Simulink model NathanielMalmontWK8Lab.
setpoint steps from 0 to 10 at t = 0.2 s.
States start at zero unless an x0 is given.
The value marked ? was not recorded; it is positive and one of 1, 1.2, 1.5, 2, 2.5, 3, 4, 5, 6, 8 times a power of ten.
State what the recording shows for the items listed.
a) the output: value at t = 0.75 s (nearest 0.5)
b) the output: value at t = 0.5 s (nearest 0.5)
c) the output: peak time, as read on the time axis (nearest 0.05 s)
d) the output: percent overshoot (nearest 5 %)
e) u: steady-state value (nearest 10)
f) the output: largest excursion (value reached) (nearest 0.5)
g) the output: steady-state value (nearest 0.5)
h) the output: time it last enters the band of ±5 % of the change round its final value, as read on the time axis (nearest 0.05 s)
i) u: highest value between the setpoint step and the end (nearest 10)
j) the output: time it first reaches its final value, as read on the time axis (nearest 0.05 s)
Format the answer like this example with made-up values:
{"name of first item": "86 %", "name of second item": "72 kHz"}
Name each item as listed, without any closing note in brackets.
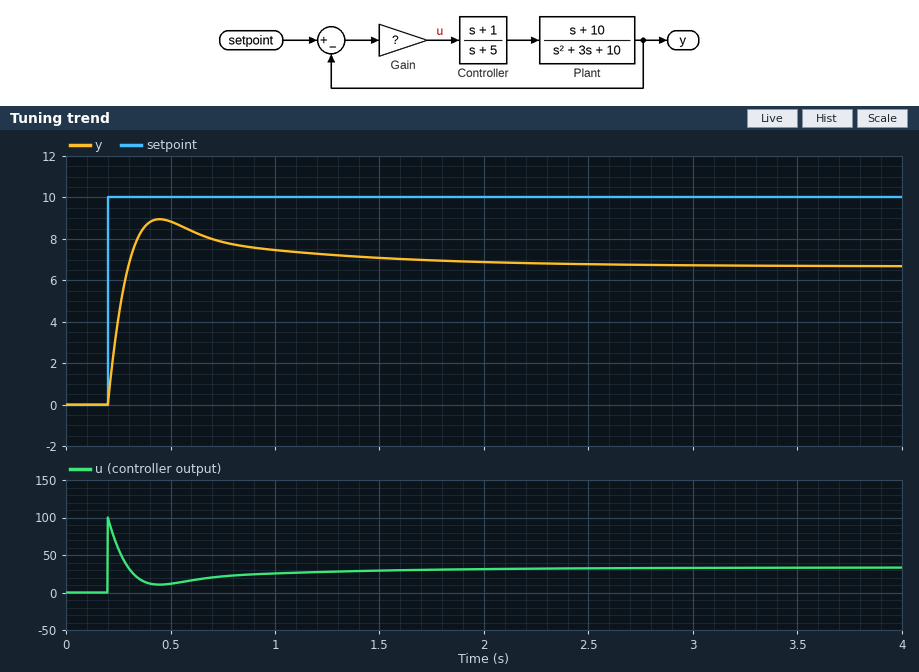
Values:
{"the output: value at t = 0.75 s": "8.0", "the output: value at t = 0.5 s": "9.0", "the output: peak time, as read on the time axis": "0.45 s", "the output: percent overshoot": "35 %", "u: steady-state value": "30", "the output: largest excursion (value reached)": "9.0", "the output: steady-state value": "6.5", "the output: time it last enters the band of ±5 % of the change round its final value, as read on the time axis": "1.65 s", "u: highest value between the setpoint step and the end": "100", "the output: time it first reaches its final value, as read on the time axis": "0.30 s"}
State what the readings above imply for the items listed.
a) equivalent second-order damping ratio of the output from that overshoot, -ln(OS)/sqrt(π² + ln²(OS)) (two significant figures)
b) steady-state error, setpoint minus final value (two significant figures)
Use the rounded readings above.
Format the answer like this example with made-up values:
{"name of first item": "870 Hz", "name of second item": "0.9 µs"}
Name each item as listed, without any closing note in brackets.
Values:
{"equivalent second-order damping ratio of the output from that overshoot, -ln(OS)/sqrt(π² + ln²(OS))": "0.32", "steady-state error, setpoint minus final value": "3.5"}
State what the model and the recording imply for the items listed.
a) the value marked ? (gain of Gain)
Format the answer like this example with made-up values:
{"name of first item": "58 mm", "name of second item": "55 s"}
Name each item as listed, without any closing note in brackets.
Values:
{"the value marked ?": "10"}
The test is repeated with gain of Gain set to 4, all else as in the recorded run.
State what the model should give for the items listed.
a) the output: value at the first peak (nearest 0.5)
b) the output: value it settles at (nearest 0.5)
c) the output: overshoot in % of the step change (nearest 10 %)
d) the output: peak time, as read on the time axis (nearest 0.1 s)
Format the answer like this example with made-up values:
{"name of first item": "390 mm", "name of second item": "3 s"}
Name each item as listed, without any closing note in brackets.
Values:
{"the output: value at the first peak": "7.0", "the output: value it settles at": "4.5", "the output: overshoot in % of the step change": "60 %", "the output: peak time, as read on the time axis": "0.6 s"}
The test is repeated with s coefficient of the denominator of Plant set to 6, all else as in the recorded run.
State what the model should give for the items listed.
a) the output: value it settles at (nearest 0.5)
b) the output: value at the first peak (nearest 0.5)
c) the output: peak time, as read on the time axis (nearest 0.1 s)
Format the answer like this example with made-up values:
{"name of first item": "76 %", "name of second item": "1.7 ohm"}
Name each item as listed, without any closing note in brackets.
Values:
{"the output: value it settles at": "6.5", "the output: value at the first peak": "8.0", "the output: peak time, as read on the time axis": "0.5 s"}
